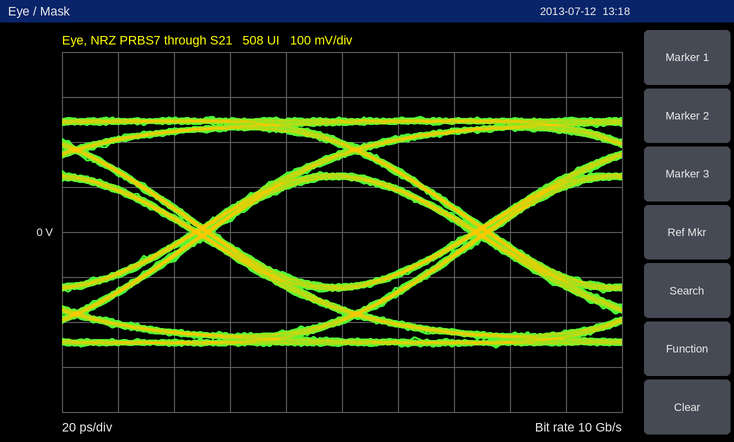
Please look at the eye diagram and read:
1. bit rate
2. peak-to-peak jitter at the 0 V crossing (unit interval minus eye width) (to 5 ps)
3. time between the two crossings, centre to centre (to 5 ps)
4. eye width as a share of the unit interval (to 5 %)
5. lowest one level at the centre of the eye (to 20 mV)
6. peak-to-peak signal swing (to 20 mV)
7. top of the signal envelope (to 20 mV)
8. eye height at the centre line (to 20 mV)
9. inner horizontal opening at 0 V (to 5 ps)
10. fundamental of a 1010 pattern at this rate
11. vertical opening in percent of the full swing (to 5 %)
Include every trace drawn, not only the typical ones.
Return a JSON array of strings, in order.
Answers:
["10 Gb/s", "10 ps", "100 ps", "90 %", "120 mV", "520 mV", "260 mV", "240 mV", "90 ps", "5 GHz", "45 %"]
